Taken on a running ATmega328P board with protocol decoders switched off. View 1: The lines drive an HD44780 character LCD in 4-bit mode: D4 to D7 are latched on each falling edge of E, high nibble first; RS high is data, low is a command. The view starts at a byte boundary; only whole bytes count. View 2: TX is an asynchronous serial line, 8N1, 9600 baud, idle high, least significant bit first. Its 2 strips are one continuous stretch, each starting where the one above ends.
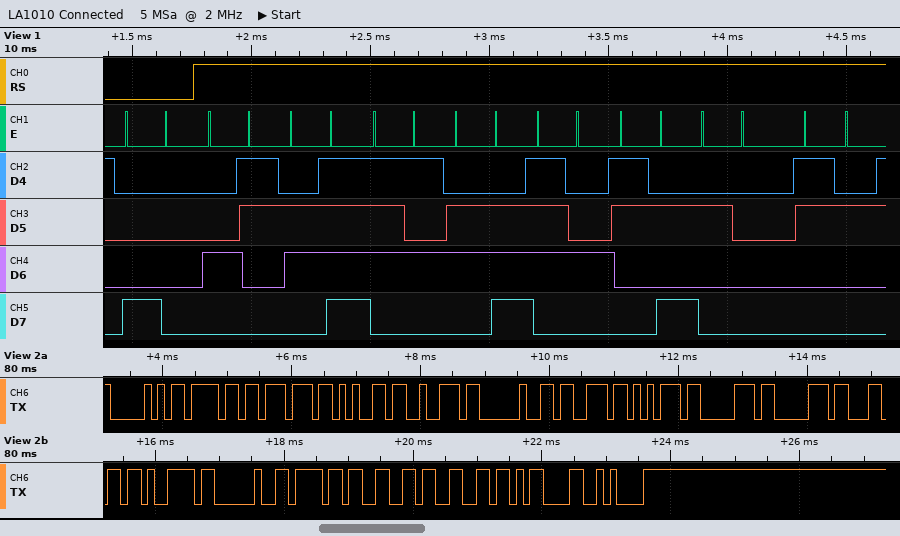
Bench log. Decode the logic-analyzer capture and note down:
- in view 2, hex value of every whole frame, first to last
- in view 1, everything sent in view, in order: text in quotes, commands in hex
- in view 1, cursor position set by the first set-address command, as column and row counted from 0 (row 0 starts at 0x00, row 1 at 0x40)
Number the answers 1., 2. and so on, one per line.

1. 50 6F 77 65 72 20 73 75 70 70 6C 79 20 6F 66 66 0D 0A
2. 0x80 "Count: 2"
3. column 0, row 0
